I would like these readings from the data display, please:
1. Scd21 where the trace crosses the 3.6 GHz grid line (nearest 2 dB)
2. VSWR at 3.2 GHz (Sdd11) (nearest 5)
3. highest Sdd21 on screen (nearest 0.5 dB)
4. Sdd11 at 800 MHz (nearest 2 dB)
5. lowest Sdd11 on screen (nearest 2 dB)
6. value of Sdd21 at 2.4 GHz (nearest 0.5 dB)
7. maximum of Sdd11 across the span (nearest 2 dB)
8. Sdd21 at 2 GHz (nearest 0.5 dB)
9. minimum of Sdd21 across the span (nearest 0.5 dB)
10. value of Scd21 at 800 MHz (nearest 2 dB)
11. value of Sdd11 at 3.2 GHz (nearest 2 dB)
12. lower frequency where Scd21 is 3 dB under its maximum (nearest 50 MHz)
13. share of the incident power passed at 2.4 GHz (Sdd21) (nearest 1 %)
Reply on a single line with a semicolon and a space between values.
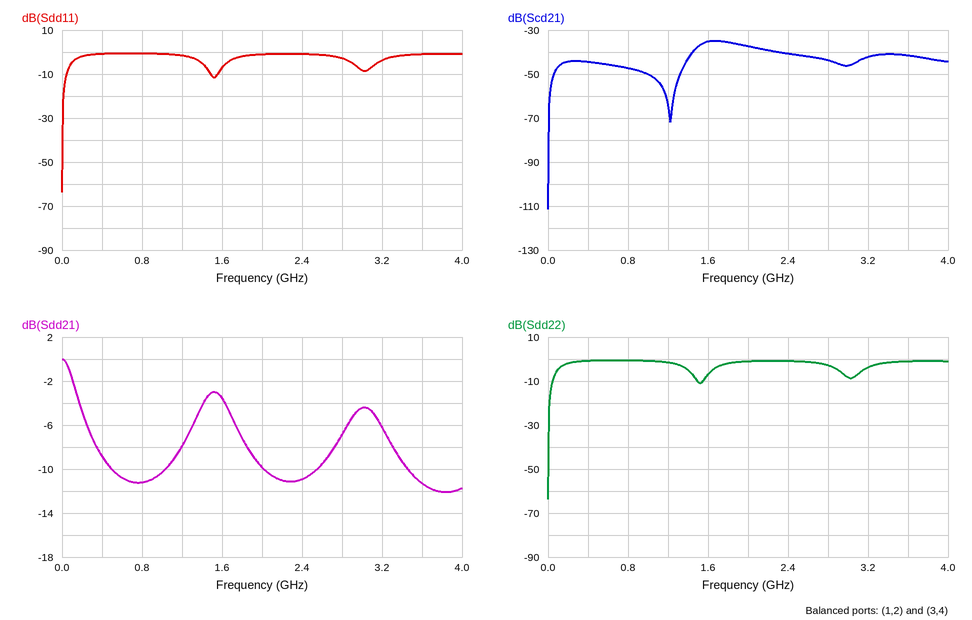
-42 dB; 5; 0.0 dB; 0 dB; -64 dB; -11.0 dB; 0 dB; -10.0 dB; -12.0 dB; -48 dB; -4 dB; 1.50 GHz; 8 %
